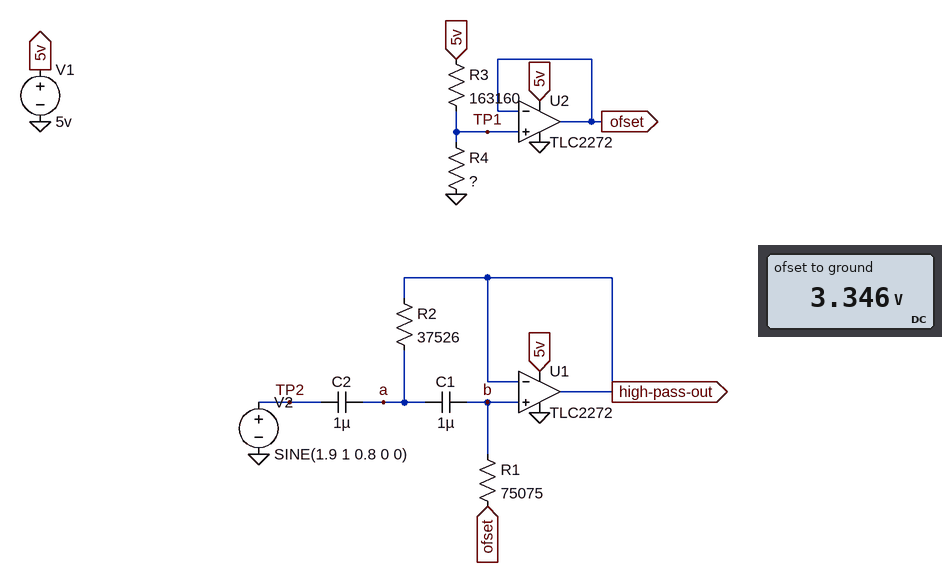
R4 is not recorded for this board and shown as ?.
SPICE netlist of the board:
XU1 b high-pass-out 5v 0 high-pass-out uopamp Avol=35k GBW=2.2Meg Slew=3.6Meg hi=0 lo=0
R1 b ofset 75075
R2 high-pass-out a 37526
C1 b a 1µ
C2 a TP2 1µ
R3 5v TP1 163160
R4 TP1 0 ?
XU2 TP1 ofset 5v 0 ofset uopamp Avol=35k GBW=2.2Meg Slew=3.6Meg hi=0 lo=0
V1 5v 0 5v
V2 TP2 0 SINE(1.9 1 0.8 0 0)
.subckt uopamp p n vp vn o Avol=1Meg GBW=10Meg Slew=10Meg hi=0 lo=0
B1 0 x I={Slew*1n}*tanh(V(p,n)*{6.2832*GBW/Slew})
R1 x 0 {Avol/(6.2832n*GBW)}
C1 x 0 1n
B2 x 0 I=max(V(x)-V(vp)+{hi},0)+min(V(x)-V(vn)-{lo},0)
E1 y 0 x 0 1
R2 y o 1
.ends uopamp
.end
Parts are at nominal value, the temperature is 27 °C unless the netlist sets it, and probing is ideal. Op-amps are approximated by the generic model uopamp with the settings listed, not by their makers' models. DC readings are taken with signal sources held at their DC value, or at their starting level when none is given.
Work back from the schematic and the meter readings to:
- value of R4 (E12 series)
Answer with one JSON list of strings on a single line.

["330 kΩ"]
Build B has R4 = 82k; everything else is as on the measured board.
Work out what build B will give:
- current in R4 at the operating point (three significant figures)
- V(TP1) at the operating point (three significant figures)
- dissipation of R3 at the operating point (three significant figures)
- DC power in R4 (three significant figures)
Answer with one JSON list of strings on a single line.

["20.4 µA", "1.67 V", "67.9 µW", "34.1 µW"]
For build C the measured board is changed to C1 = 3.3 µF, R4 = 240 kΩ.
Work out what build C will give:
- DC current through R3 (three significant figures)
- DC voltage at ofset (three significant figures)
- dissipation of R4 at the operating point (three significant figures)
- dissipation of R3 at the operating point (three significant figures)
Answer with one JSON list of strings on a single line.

["12.4 µA", "2.98 V", "36.9 µW", "25.1 µW"]
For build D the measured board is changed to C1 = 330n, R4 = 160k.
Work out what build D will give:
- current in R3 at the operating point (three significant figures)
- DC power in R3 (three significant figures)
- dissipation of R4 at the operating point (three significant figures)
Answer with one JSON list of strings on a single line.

["15.5 µA", "39.1 µW", "38.3 µW"]
